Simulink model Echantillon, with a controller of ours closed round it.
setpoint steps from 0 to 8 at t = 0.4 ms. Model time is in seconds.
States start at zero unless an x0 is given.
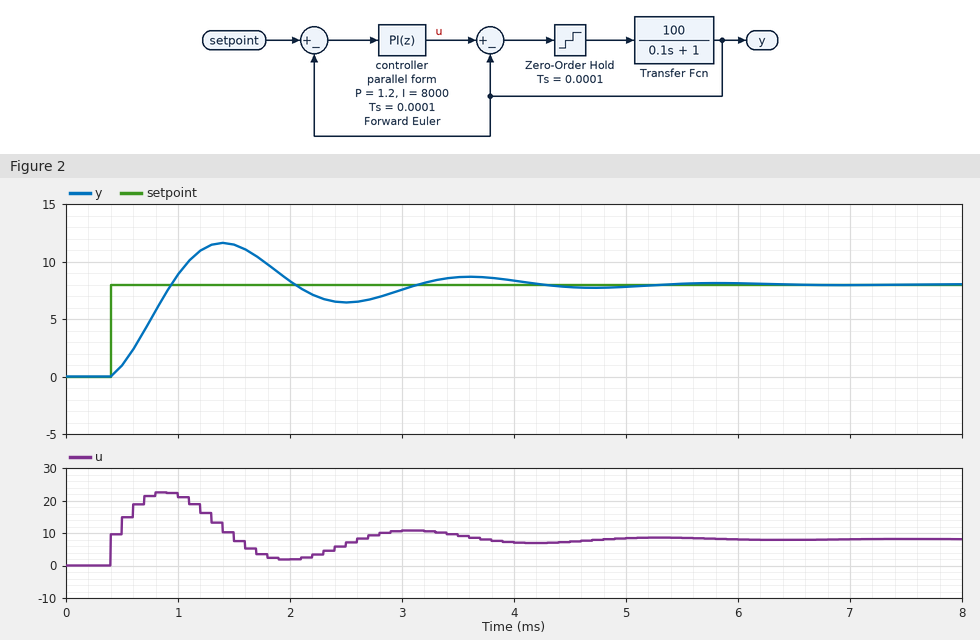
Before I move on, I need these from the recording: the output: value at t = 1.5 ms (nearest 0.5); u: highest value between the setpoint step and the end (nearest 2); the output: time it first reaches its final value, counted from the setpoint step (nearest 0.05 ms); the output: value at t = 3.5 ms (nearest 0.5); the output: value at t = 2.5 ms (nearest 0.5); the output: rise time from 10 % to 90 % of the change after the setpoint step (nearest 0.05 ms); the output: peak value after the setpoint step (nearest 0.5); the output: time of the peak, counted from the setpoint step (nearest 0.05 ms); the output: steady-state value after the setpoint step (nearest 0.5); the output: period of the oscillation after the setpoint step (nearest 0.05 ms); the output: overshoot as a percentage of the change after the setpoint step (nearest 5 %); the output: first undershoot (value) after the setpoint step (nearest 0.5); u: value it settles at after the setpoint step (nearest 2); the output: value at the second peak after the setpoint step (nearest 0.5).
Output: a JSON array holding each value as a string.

["11.5", "22", "0.55 ms", "8.5", "6.5", "0.40 ms", "11.5", "1.00 ms", "8.0", "2.20 ms", "45 %", "6.5", "8", "8.5"]
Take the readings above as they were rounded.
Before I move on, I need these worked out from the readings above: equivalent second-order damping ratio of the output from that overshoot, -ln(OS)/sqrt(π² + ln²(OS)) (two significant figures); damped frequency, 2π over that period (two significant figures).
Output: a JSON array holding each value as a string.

["0.25", "2.9 rad/ms"]
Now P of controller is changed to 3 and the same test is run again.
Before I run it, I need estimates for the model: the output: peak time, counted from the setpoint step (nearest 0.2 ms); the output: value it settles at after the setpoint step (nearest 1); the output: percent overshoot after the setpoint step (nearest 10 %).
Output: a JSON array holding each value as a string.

["0.8 ms", "8", "20 %"]
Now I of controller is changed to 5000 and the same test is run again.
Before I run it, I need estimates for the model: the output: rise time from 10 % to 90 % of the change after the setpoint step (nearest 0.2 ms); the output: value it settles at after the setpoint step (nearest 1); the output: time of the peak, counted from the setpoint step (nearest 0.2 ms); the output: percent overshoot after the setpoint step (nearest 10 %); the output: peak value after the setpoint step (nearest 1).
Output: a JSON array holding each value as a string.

["0.6 ms", "8", "1.2 ms", "30 %", "10"]
